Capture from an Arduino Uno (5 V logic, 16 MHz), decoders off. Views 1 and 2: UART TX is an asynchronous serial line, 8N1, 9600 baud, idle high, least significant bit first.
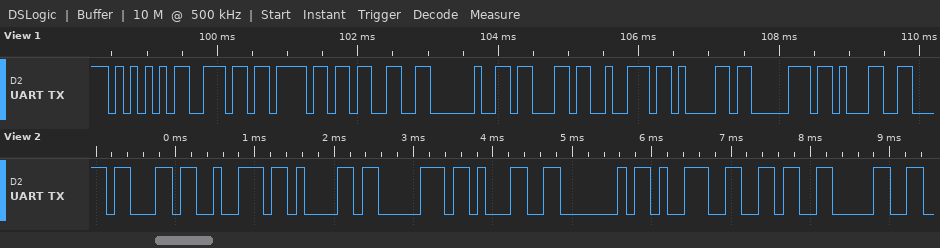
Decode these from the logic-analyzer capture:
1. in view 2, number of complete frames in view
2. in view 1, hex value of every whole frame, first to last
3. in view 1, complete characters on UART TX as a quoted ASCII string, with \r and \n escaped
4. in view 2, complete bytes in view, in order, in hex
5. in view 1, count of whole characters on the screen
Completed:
9
55 6E 6F 33 20 63 72 61 70 31
"Uno3 crap1"
63 72 61 70 31 40 39 36 30
10
